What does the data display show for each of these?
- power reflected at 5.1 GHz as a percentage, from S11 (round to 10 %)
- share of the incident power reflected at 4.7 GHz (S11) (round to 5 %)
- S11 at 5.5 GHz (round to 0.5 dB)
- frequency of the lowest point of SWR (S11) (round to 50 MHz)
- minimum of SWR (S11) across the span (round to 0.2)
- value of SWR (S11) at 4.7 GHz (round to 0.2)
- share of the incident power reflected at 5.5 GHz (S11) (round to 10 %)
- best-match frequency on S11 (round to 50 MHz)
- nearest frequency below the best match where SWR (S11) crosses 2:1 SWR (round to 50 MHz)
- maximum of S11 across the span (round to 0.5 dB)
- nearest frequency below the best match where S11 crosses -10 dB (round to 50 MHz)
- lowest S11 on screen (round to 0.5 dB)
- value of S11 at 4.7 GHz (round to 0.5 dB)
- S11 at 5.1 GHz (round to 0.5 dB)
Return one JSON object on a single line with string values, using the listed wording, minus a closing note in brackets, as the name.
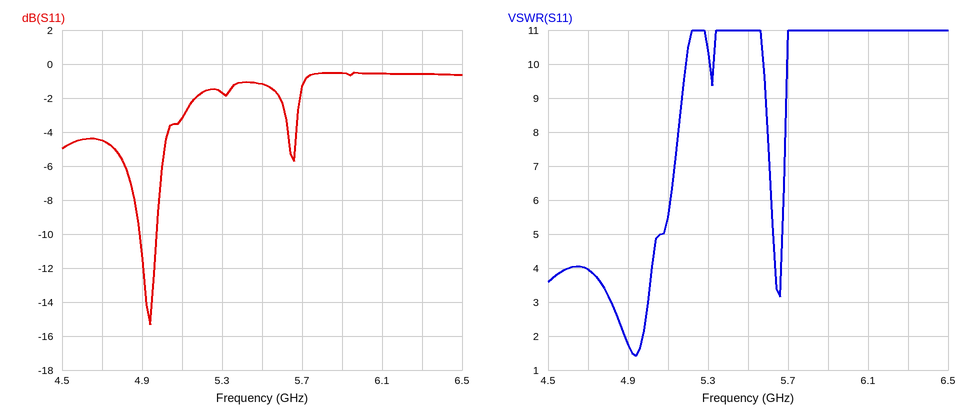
{"power reflected at 5.1 GHz as a percentage, from S11": "50 %", "share of the incident power reflected at 4.7 GHz (S11)": "35 %", "S11 at 5.5 GHz": "-1.0 dB", "frequency of the lowest point of SWR (S11)": "4.95 GHz", "minimum of SWR (S11) across the span": "1.4", "value of SWR (S11) at 4.7 GHz": "4.0", "share of the incident power reflected at 5.5 GHz (S11)": "80 %", "best-match frequency on S11": "4.95 GHz", "nearest frequency below the best match where SWR (S11) crosses 2:1 SWR": "4.90 GHz", "maximum of S11 across the span": "-0.5 dB", "nearest frequency below the best match where S11 crosses -10 dB": "4.90 GHz", "lowest S11 on screen": "-15.5 dB", "value of S11 at 4.7 GHz": "-4.5 dB", "S11 at 5.1 GHz": "-3.0 dB"}
